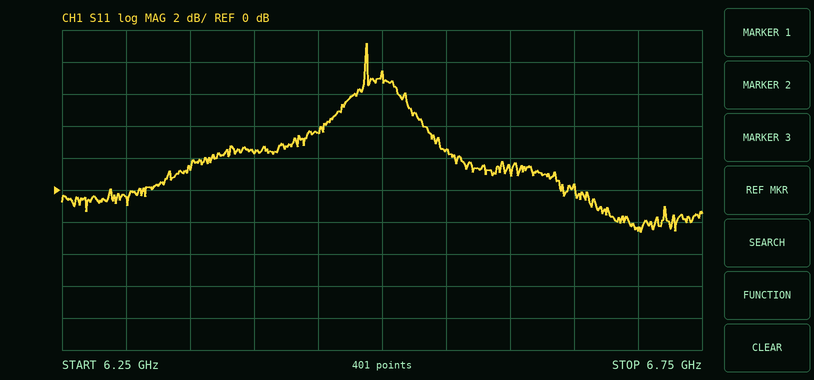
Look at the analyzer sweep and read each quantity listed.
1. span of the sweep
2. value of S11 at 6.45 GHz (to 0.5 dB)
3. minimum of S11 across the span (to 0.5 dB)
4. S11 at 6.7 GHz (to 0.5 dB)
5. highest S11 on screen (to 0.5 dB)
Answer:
500 MHz
3.5 dB
-2.5 dB
-2.5 dB
9.0 dB
